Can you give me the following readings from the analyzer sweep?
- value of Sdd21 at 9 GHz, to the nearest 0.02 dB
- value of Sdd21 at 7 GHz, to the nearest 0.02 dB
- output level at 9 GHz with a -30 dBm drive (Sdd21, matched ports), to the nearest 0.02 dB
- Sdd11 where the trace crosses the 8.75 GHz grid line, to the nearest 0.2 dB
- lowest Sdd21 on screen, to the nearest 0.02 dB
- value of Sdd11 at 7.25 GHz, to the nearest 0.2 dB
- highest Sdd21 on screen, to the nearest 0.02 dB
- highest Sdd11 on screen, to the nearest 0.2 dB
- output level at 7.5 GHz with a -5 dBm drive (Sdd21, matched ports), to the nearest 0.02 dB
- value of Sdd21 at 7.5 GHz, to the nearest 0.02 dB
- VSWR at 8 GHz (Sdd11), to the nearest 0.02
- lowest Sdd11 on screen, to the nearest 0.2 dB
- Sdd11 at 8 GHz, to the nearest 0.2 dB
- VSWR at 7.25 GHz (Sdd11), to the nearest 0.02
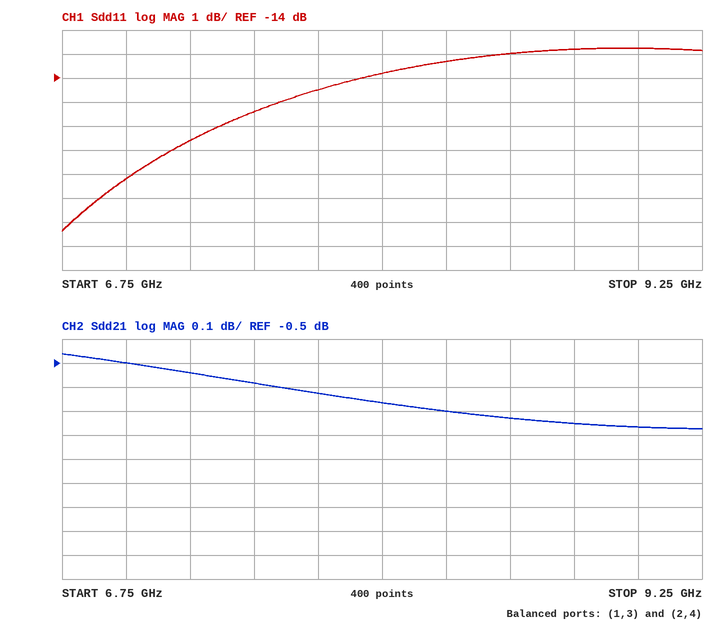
-0.76 dB
-0.50 dB
-30.76 dBm
-12.8 dB
-0.78 dB
-16.6 dB
-0.46 dB
-12.8 dB
-5.58 dBm
-0.58 dB
1.52
-20.4 dB
-13.8 dB
1.34
